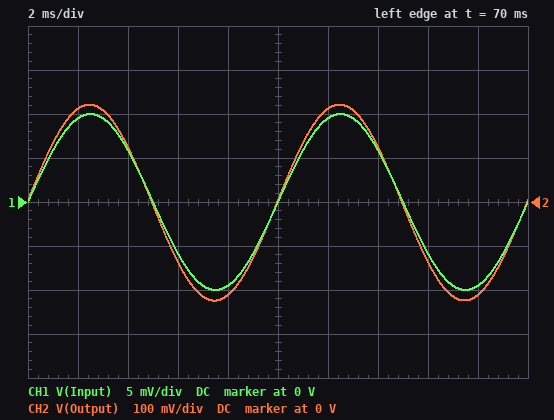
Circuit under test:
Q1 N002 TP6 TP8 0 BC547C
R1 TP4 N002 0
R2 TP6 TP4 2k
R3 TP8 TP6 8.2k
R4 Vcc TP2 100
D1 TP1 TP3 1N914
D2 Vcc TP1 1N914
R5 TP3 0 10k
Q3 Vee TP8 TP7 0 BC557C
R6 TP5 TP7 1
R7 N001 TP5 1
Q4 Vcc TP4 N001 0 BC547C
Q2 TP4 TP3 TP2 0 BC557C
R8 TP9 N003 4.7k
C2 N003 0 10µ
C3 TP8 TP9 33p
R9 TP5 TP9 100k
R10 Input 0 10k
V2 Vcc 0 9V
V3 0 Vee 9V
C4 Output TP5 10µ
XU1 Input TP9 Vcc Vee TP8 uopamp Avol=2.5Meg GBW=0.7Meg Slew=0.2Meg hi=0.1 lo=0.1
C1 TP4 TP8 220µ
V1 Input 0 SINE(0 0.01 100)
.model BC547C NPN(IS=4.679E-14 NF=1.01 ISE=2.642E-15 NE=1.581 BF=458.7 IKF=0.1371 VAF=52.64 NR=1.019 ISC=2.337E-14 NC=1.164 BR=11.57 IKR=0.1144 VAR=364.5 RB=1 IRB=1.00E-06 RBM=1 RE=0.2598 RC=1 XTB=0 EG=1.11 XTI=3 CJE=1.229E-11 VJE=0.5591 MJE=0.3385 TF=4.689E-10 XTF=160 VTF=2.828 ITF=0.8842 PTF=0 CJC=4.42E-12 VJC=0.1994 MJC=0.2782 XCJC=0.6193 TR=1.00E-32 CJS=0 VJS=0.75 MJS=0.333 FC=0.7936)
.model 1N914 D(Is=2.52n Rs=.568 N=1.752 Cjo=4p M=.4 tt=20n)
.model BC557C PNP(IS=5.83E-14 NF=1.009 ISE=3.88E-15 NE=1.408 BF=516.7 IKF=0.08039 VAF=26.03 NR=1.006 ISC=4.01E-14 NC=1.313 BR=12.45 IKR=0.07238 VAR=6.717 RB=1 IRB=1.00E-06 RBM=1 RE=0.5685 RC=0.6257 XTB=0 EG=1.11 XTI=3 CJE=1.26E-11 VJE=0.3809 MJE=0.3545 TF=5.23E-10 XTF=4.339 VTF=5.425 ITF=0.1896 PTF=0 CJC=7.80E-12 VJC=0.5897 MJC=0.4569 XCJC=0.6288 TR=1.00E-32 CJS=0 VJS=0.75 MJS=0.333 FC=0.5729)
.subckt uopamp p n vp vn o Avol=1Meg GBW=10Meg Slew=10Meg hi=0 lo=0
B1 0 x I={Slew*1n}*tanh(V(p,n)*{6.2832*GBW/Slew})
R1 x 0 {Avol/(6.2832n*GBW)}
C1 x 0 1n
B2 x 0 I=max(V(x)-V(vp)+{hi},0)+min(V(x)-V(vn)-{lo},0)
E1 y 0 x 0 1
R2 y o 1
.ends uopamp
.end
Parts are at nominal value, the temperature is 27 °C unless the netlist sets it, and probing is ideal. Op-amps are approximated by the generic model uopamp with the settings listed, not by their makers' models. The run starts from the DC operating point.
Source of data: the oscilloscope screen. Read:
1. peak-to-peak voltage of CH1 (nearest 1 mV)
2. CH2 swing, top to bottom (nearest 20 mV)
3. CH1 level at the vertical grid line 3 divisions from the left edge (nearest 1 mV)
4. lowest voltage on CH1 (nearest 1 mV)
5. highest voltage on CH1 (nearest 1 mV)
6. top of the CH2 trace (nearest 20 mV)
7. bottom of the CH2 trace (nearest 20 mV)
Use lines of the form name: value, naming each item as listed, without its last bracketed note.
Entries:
peak-to-peak voltage of CH1: 20 mV
CH2 swing, top to bottom: 440 mV
CH1 level at the vertical grid line 3 divisions from the left edge: -6 mV
lowest voltage on CH1: -10 mV
highest voltage on CH1: 10 mV
top of the CH2 trace: 220 mV
bottom of the CH2 trace: -220 mV
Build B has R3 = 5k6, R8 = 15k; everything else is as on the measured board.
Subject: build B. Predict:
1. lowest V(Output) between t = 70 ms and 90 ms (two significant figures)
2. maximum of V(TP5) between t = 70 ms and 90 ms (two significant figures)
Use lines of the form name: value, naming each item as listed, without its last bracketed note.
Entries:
lowest V(Output) between t = 70 ms and 90 ms: -77 mV
maximum of V(TP5) between t = 70 ms and 90 ms: 76 mV
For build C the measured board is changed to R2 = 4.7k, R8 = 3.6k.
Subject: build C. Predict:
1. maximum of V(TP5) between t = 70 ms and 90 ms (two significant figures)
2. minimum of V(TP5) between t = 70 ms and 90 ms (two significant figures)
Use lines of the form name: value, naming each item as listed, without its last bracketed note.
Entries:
maximum of V(TP5) between t = 70 ms and 90 ms: 290 mV
minimum of V(TP5) between t = 70 ms and 90 ms: -290 mV
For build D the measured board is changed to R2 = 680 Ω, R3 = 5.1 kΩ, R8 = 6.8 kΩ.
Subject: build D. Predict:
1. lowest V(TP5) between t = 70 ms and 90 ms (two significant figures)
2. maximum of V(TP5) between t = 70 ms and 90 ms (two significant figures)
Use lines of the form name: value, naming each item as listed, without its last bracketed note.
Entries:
lowest V(TP5) between t = 70 ms and 90 ms: -160 mV
maximum of V(TP5) between t = 70 ms and 90 ms: 160 mV
